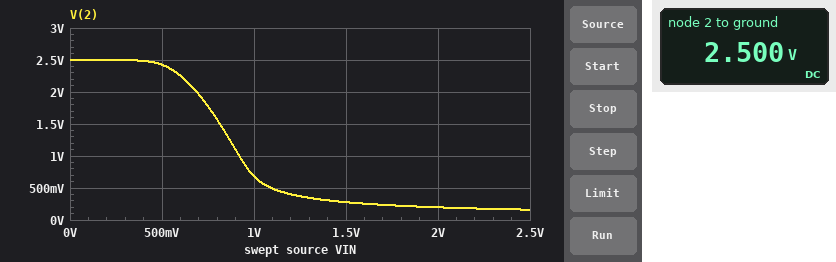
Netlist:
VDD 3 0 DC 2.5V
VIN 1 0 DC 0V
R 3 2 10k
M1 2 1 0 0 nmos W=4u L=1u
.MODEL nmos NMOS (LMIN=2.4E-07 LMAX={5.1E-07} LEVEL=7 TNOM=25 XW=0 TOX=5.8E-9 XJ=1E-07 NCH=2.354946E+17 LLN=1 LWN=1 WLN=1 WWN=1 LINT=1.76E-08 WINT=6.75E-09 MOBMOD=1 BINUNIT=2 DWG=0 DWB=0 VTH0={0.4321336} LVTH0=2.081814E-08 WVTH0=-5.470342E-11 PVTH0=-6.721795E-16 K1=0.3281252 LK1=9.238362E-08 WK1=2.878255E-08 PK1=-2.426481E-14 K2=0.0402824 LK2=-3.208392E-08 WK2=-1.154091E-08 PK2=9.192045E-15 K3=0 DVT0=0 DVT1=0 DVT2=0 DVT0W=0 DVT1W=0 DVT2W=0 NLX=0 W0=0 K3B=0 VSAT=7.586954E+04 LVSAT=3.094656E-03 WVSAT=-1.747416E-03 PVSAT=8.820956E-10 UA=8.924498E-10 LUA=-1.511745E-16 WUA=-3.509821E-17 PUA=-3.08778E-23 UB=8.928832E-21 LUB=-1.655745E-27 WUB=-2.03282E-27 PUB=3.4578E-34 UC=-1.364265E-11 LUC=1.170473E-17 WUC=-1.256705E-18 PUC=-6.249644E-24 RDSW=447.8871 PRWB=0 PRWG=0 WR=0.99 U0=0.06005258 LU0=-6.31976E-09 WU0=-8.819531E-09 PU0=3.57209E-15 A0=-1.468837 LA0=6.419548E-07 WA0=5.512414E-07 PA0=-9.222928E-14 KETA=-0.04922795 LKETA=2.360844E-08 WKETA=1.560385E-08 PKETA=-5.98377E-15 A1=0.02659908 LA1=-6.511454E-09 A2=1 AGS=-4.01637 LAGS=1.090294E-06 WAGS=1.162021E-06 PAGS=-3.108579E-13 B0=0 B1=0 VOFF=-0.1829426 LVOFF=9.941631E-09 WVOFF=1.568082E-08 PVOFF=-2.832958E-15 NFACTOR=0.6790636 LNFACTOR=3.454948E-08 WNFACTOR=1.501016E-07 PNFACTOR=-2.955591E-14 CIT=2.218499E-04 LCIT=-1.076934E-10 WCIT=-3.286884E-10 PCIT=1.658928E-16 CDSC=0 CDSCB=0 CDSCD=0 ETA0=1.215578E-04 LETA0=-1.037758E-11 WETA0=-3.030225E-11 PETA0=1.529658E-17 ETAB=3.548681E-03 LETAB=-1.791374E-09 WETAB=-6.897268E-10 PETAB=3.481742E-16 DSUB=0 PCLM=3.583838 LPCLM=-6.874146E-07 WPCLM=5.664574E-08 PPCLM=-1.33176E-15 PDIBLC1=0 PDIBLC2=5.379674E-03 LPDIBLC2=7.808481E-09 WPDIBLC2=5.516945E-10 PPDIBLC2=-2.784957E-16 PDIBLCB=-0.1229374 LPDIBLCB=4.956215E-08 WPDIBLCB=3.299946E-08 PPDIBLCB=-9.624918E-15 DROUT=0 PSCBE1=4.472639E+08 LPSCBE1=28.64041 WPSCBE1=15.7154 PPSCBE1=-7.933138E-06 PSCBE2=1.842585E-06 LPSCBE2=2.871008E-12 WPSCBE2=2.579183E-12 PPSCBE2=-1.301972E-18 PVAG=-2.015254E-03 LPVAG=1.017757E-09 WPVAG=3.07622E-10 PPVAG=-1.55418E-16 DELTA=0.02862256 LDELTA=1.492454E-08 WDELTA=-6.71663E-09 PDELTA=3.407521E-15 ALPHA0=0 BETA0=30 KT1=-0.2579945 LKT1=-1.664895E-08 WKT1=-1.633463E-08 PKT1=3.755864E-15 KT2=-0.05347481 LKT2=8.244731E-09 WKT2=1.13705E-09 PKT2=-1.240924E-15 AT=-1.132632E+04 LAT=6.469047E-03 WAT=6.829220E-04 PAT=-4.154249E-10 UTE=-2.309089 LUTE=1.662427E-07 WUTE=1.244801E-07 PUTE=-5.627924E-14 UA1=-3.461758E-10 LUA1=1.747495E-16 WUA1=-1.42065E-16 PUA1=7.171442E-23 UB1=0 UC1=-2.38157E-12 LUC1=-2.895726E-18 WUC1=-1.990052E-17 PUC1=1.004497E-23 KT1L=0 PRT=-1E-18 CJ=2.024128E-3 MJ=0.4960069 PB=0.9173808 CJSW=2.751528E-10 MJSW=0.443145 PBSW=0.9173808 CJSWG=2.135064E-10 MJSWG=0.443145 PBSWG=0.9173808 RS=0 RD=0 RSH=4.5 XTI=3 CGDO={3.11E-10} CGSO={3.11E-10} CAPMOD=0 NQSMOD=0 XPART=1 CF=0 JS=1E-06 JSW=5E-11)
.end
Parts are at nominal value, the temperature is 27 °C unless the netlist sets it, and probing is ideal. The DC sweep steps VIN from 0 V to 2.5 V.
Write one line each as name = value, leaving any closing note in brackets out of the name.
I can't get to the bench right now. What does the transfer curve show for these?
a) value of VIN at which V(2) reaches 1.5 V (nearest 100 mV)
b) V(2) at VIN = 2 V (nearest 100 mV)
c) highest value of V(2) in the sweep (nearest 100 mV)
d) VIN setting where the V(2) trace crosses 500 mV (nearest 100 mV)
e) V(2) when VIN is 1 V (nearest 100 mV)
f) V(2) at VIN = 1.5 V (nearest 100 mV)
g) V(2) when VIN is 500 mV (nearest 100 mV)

value of VIN at which V(2) reaches 1.5 V = 800 mV
V(2) at VIN = 2 V = 200 mV
highest value of V(2) in the sweep = 2.5 V
VIN setting where the V(2) trace crosses 500 mV = 1.1 V
V(2) when VIN is 1 V = 700 mV
V(2) at VIN = 1.5 V = 300 mV
V(2) when VIN is 500 mV = 2.4 V
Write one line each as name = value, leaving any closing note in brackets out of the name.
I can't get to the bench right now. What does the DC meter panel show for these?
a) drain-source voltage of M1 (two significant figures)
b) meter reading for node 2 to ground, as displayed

drain-source voltage of M1 = 2.5 V
meter reading for node 2 to ground, as displayed = 2.500 V
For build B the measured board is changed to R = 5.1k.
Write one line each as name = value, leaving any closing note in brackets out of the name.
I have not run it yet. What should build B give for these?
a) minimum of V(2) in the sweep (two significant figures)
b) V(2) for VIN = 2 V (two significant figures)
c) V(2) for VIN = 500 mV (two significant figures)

minimum of V(2) in the sweep = 310 mV
V(2) for VIN = 2 V = 380 mV
V(2) for VIN = 500 mV = 2.5 V
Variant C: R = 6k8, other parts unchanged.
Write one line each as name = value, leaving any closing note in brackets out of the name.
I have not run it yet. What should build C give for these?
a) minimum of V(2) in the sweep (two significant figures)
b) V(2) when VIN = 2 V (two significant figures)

minimum of V(2) in the sweep = 230 mV
V(2) when VIN = 2 V = 290 mV
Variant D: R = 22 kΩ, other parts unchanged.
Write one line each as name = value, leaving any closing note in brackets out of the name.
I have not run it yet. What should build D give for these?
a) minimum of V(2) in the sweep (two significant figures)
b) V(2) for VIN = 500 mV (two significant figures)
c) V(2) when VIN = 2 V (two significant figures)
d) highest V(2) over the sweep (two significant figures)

minimum of V(2) in the sweep = 74 mV
V(2) for VIN = 500 mV = 2.3 V
V(2) when VIN = 2 V = 91 mV
highest V(2) over the sweep = 2.5 V
